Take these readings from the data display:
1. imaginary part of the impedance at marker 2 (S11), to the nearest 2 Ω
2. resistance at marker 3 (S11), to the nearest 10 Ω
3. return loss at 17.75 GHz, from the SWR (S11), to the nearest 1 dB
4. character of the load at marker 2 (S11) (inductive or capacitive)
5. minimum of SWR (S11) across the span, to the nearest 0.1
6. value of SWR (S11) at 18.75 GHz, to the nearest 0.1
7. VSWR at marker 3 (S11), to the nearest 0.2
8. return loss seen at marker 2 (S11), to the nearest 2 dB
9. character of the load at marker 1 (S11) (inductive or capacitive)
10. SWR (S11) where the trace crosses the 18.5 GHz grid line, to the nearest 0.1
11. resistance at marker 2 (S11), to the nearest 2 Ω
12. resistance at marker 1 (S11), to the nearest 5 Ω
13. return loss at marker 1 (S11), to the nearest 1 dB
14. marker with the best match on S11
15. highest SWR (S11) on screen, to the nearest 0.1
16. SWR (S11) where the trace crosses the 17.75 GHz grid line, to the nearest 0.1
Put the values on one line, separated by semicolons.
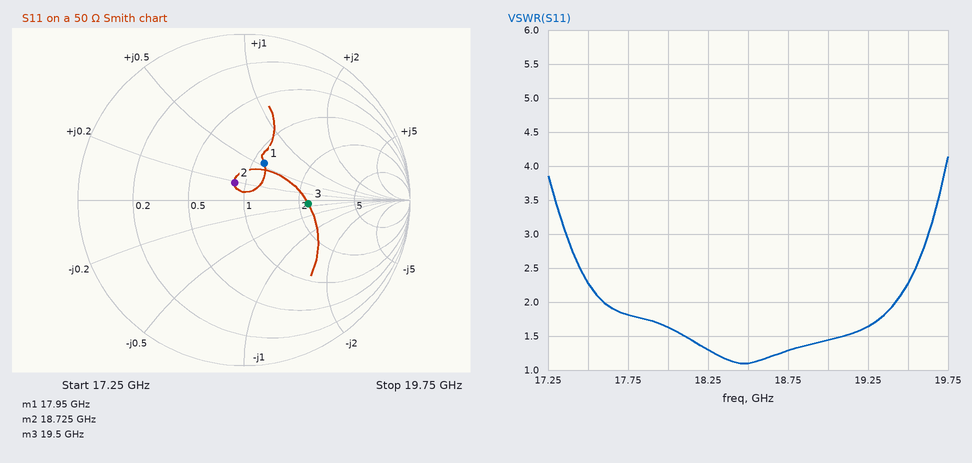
+10 Ω; 110 Ω; 11 dB; inductive; 1.1; 1.3; 2.2; 18 dB; inductive; 1.1; 44 Ω; 55 Ω; 12 dB; marker 2; 4.1; 1.8
